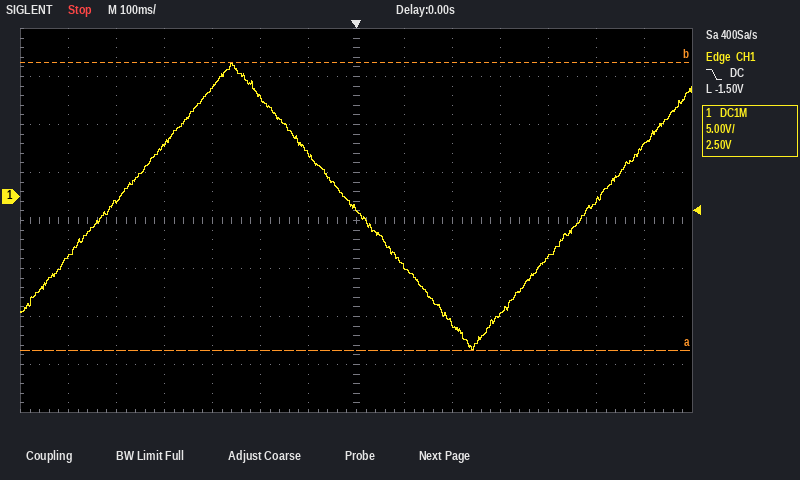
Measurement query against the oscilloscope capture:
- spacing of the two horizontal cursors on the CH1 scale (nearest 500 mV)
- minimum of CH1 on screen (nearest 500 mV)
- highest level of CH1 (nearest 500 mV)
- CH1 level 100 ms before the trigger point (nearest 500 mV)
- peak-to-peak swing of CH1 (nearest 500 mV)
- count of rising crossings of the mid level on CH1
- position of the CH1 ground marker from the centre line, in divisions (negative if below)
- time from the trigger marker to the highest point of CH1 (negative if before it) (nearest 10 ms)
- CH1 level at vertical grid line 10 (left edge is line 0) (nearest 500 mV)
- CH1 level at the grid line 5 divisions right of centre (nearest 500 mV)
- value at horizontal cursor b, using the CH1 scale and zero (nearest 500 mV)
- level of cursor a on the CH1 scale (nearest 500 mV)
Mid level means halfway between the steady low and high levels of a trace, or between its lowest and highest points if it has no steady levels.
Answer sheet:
30.0 V
-16.0 V
14.0 V
4.5 V
30.0 V
2
+0.5 div
-260 ms
-12.5 V
-500 mV
14.0 V
-16.0 V
